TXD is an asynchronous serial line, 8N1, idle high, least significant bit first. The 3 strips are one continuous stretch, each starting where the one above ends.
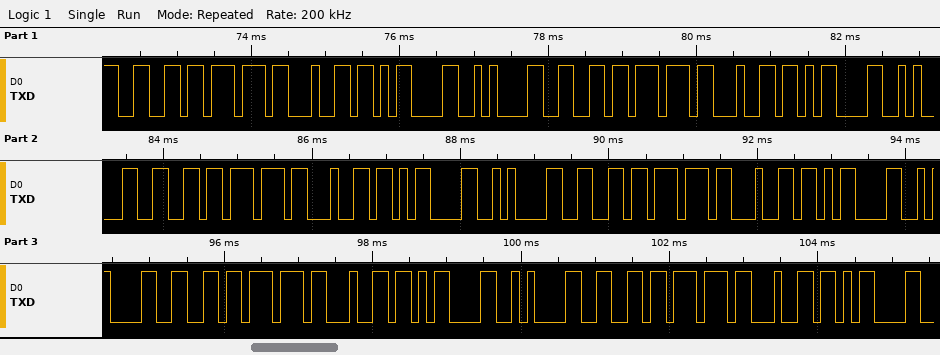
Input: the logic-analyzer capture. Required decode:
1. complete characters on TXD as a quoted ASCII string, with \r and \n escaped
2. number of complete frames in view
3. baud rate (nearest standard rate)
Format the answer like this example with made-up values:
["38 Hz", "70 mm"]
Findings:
["\"fwd\\r\\nfwd\\r\\nfwd\\r\\nfwd\\r\\nfwd\\r\\nfwd\\r\"", "29", "9600 baud"]
